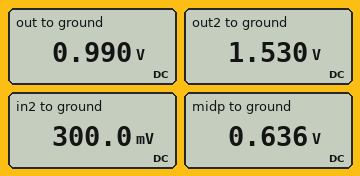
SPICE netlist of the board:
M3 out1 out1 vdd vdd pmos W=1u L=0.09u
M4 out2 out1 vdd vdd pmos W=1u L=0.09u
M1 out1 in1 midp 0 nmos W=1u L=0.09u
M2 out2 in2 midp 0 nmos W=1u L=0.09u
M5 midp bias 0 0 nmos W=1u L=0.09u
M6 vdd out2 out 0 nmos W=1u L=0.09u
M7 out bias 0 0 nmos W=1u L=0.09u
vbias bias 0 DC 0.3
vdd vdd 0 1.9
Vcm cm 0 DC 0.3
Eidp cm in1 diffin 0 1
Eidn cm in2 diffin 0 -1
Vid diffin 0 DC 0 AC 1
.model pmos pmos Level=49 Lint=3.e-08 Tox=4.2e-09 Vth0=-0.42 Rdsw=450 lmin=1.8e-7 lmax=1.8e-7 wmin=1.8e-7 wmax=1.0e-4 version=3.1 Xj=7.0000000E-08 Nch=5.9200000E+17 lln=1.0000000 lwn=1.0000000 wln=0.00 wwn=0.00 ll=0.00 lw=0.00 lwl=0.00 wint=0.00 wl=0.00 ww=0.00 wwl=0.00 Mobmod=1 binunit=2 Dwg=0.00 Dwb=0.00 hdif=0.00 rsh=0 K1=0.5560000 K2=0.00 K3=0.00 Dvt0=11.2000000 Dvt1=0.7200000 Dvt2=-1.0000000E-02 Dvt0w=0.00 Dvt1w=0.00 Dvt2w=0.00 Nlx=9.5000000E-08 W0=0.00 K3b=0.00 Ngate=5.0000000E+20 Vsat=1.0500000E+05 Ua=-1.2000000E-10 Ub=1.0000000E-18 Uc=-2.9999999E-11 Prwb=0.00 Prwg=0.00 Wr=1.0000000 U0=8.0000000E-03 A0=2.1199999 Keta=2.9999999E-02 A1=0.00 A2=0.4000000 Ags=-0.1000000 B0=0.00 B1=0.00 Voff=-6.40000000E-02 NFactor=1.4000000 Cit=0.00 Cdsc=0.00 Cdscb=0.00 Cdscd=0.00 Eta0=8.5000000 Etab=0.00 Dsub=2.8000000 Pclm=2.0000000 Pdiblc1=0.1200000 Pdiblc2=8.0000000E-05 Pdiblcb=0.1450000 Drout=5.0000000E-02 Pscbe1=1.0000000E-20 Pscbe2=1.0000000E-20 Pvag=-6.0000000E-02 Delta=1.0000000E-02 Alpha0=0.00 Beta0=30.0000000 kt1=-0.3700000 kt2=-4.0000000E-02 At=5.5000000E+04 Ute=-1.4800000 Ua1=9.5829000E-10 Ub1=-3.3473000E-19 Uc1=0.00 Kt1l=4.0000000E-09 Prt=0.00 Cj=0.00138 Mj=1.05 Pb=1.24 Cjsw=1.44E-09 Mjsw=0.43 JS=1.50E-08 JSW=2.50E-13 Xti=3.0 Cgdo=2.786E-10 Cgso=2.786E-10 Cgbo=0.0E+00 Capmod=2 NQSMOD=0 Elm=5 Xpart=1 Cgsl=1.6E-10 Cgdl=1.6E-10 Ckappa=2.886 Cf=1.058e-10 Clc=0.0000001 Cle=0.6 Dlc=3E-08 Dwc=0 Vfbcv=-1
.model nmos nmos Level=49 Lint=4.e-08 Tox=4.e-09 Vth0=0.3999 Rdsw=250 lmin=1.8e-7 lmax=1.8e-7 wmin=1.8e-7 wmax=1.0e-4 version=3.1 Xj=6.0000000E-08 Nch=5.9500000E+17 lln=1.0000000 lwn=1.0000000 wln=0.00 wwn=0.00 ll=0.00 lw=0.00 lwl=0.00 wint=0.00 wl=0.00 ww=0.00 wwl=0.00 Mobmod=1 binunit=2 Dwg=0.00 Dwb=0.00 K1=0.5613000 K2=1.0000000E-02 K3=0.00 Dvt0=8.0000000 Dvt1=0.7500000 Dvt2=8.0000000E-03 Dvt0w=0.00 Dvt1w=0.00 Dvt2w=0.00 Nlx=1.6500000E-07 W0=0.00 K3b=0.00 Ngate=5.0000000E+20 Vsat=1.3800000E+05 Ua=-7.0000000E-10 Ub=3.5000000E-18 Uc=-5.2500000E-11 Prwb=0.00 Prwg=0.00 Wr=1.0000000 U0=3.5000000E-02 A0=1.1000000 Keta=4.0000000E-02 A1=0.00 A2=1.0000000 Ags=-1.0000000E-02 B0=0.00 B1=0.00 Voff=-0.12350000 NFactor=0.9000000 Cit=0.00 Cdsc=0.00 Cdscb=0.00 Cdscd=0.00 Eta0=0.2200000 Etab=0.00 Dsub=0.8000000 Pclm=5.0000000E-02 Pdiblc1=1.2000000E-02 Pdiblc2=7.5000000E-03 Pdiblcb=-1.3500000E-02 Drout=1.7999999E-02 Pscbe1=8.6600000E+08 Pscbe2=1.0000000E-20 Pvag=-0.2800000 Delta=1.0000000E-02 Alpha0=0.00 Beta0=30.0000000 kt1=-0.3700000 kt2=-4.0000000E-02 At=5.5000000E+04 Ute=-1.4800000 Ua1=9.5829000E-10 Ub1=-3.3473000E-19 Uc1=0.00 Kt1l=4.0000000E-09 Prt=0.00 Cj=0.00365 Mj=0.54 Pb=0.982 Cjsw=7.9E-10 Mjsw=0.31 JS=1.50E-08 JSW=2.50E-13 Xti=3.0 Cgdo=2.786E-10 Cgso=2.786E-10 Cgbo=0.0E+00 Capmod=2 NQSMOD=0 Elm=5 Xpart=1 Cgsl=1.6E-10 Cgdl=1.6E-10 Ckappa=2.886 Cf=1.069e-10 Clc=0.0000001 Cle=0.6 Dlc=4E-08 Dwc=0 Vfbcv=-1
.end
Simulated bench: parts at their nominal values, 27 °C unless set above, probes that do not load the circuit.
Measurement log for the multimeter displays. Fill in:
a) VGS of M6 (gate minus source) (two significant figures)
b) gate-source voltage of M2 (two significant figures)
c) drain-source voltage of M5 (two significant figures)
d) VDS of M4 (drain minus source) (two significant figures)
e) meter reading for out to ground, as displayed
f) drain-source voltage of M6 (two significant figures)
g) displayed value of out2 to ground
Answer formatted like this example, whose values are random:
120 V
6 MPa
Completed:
540 mV
-340 mV
640 mV
-370 mV
0.990 V
910 mV
1.530 V
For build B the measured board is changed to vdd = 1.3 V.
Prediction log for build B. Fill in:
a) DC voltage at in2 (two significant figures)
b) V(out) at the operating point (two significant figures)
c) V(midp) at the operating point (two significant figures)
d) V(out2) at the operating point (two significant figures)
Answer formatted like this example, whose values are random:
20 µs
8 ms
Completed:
300 mV
630 mV
480 mV
980 mV
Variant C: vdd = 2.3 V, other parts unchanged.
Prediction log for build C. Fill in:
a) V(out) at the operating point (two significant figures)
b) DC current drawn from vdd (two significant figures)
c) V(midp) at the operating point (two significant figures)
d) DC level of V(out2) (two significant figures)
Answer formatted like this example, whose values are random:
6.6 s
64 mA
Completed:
1.2 V
2.3 mA
730 mV
1.9 V
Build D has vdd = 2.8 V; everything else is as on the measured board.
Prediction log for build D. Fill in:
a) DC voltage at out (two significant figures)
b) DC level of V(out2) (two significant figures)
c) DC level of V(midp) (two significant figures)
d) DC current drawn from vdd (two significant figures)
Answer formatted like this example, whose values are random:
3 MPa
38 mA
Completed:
1.5 V
2.4 V
850 mV
2.7 mA
